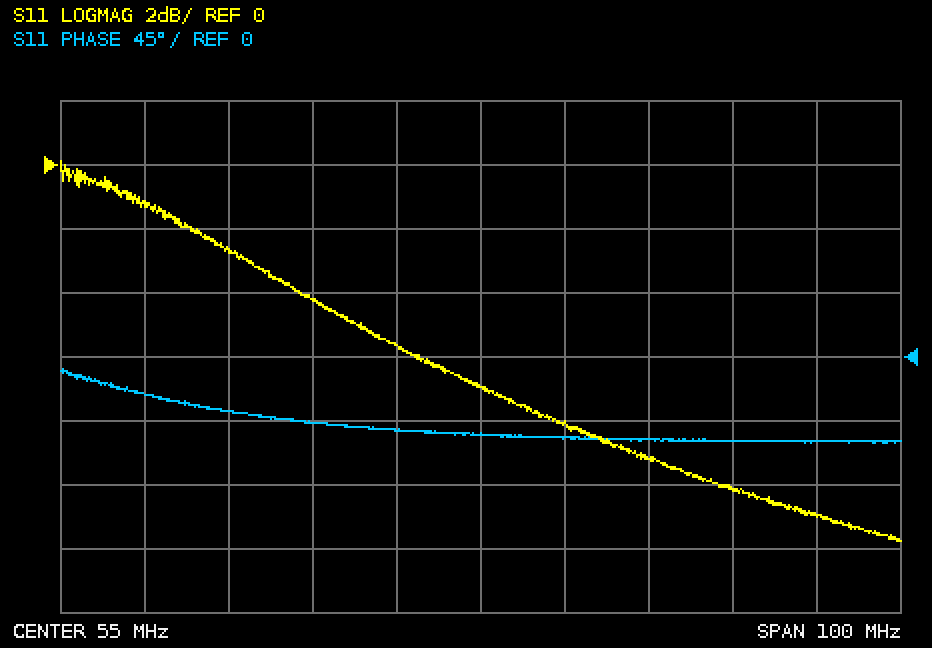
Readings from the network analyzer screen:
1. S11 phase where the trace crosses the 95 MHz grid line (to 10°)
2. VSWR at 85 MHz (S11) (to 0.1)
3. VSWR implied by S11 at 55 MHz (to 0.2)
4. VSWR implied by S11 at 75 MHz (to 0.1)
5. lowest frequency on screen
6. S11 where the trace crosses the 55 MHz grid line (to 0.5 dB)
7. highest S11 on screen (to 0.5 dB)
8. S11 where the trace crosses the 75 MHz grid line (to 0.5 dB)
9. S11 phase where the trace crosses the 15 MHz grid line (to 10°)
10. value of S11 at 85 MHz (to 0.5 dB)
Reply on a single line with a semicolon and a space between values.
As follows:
-60°; 1.9; 2.6; 2.1; 5 MHz; -7.0 dB; 0.0 dB; -9.0 dB; -30°; -10.0 dB
